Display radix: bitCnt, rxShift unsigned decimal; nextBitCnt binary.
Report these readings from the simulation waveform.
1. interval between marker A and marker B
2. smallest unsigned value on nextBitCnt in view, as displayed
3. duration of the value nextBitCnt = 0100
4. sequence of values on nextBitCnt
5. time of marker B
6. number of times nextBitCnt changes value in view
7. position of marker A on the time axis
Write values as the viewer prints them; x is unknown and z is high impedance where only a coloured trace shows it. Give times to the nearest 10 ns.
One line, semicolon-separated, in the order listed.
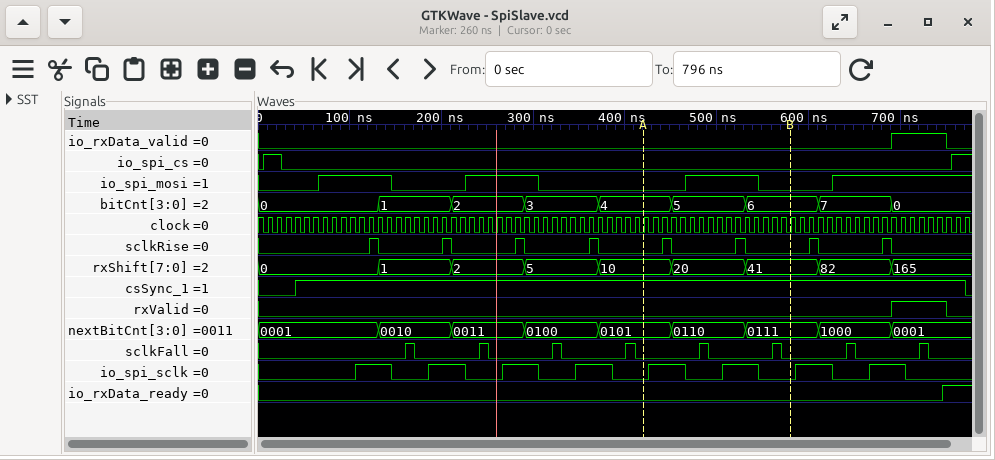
160 ns; 0001; 80 ns; 0001, 0010, 0011, 0100, 0101, 0110, 0111, 1000, 0001; 580 ns; 8; 420 ns
